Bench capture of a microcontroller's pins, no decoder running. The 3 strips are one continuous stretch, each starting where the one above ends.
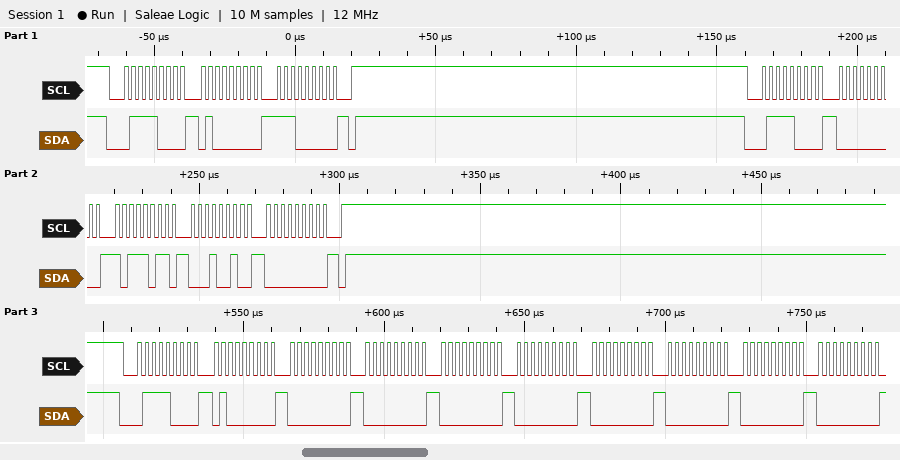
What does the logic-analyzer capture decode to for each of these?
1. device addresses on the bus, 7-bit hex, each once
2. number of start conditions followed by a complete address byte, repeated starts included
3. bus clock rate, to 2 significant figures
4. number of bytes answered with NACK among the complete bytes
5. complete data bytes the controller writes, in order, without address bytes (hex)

0x3C
3
400 kHz
0
40 E0 00 BB 12 00 40 00 00 00 00 00 00 00 00
